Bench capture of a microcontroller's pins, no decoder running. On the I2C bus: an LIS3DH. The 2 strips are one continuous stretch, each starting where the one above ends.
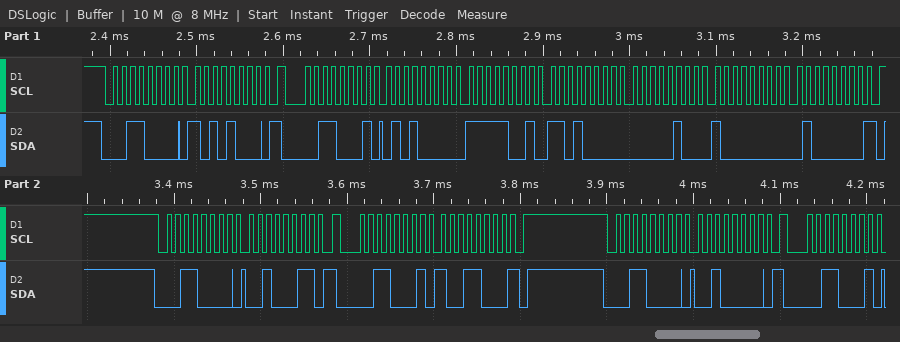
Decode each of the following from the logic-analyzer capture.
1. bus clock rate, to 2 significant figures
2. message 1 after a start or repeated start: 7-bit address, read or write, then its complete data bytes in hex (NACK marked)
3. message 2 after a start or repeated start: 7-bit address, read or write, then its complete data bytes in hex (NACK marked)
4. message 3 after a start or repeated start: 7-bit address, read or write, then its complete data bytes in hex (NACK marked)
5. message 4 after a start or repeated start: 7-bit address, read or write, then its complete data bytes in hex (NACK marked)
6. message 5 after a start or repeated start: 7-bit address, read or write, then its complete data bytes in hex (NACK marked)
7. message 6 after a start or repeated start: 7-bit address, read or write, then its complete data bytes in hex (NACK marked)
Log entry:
100 kHz
0x18 write: A8
0x18 read: 50 F9 D0 04 80 40 NACK
0x18 write: 23
0x18 read: 98 NACK
0x18 write: 20
0x18 read
